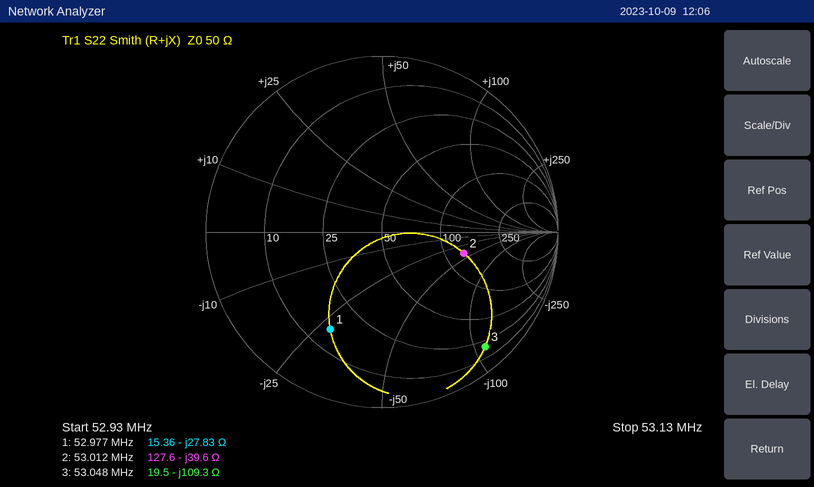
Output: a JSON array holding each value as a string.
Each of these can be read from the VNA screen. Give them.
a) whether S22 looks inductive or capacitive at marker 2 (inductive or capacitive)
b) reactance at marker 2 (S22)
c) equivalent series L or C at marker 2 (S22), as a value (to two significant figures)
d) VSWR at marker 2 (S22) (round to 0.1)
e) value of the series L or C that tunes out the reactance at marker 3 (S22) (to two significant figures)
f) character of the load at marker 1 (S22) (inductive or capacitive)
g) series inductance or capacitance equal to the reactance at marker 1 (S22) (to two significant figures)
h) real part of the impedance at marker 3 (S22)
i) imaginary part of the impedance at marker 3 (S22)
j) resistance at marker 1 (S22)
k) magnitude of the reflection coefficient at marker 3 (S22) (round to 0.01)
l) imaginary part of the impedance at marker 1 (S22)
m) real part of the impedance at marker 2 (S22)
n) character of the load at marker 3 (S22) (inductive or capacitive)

["capacitive", "-39.6 Ω", "76 pF", "2.8", "330 nH", "capacitive", "110 pF", "19.5 Ω", "-109.3 Ω", "15.36 Ω", "0.88", "-27.83 Ω", "127.6 Ω", "capacitive"]
